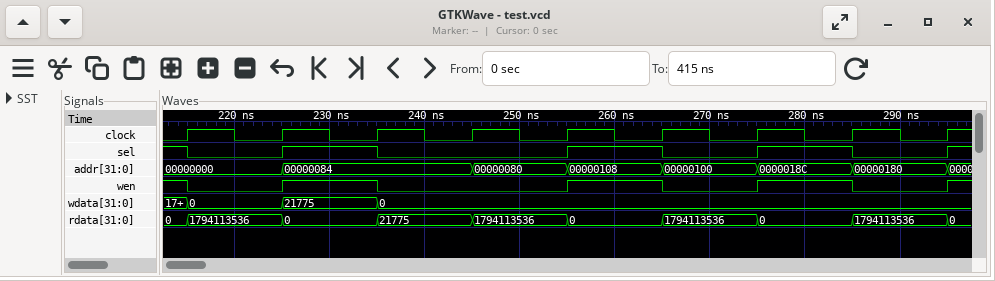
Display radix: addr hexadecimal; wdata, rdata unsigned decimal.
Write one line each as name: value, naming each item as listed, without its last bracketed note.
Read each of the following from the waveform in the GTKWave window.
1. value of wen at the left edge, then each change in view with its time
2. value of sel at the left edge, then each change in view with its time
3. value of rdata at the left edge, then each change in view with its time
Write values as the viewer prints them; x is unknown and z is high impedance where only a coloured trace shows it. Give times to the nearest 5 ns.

value of wen at the left edge, then each change in view with its time: 1, 0 at 215 ns, 1 at 225 ns, 0 at 235 ns, 1 at 255 ns, 0 at 265 ns, 1 at 275 ns, 0 at 285 ns, 1 at 295 ns
value of sel at the left edge, then each change in view with its time: 1, 0 at 215 ns, 1 at 225 ns, 0 at 235 ns, 1 at 255 ns, 0 at 265 ns, 1 at 275 ns, 0 at 285 ns, 1 at 295 ns
value of rdata at the left edge, then each change in view with its time: 0, 1794113536 at 215 ns, 0 at 225 ns, 21775 at 235 ns, 1794113536 at 245 ns, 0 at 255 ns, 1794113536 at 265 ns, 0 at 275 ns, 1794113536 at 285 ns, 0 at 295 ns
